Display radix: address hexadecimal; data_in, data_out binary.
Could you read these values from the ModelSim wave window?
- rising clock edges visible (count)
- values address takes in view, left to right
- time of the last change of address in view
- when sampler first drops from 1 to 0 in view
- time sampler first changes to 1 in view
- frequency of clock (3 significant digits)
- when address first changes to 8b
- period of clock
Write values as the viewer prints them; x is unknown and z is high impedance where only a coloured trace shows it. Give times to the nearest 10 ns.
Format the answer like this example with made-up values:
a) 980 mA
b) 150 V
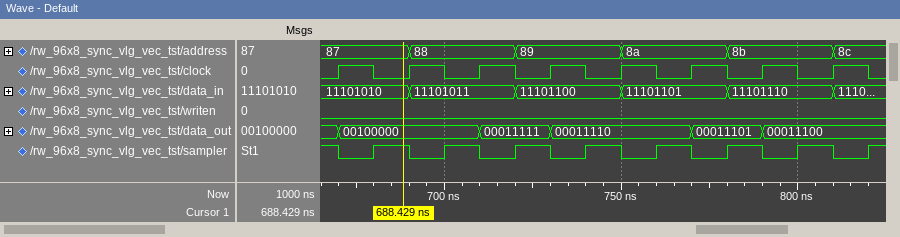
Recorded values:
a) 8
b) 87, 88, 89, 8a, 8b, 8c
c) 810 ns
d) 670 ns
e) 680 ns
f) 50.0 MHz
g) 780 ns
h) 20 ns
